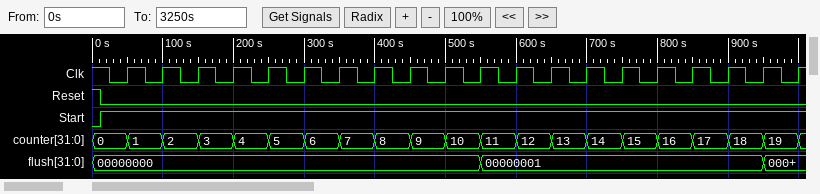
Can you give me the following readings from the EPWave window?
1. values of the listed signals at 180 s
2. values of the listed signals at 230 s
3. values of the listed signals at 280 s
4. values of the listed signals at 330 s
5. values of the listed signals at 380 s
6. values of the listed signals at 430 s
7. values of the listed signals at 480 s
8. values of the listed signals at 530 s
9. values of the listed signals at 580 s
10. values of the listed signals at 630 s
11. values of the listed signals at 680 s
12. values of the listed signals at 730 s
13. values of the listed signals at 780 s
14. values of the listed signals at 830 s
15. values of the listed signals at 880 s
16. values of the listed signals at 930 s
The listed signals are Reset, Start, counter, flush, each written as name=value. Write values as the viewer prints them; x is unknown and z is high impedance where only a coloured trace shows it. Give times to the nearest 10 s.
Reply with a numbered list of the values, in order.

1. Reset=0, Start=1, counter=3, flush=00000000
2. Reset=0, Start=1, counter=4, flush=00000000
3. Reset=0, Start=1, counter=5, flush=00000000
4. Reset=0, Start=1, counter=6, flush=00000000
5. Reset=0, Start=1, counter=7, flush=00000000
6. Reset=0, Start=1, counter=8, flush=00000000
7. Reset=0, Start=1, counter=9, flush=00000000
8. Reset=0, Start=1, counter=10, flush=00000000
9. Reset=0, Start=1, counter=11, flush=00000001
10. Reset=0, Start=1, counter=12, flush=00000001
11. Reset=0, Start=1, counter=13, flush=00000001
12. Reset=0, Start=1, counter=14, flush=00000001
13. Reset=0, Start=1, counter=15, flush=00000001
14. Reset=0, Start=1, counter=16, flush=00000001
15. Reset=0, Start=1, counter=17, flush=00000001
16. Reset=0, Start=1, counter=18, flush=00000001
